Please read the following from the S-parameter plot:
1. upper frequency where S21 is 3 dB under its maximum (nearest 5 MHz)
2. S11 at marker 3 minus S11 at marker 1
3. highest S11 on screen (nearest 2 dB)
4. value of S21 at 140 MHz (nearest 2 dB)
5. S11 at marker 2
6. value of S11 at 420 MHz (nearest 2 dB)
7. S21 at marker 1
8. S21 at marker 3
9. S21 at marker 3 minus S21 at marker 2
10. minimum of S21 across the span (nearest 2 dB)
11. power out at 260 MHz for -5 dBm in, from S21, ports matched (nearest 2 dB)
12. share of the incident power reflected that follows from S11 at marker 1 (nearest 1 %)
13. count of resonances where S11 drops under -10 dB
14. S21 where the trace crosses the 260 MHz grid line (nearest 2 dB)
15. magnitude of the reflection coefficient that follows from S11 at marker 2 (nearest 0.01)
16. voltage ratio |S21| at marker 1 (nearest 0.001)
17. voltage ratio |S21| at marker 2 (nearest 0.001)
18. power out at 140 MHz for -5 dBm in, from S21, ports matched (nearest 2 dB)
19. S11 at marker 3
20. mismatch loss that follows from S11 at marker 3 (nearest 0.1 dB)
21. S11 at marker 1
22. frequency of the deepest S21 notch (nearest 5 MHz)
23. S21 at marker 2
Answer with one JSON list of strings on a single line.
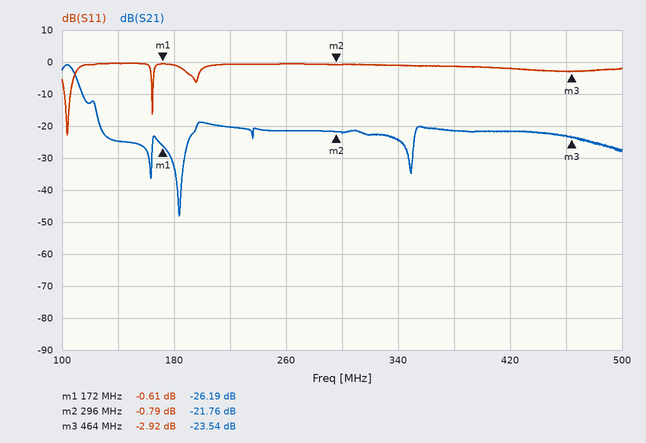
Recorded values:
["110 MHz", "-2.31 dB", "0 dB", "-24 dB", "-0.79 dB", "-2 dB", "-26.19 dB", "-23.54 dB", "-1.78 dB", "-48 dB", "-26 dBm", "87 %", "2", "-22 dB", "0.91", "0.049", "0.082", "-30 dBm", "-2.92 dB", "3.1 dB", "-0.61 dB", "185 MHz", "-21.76 dB"]
